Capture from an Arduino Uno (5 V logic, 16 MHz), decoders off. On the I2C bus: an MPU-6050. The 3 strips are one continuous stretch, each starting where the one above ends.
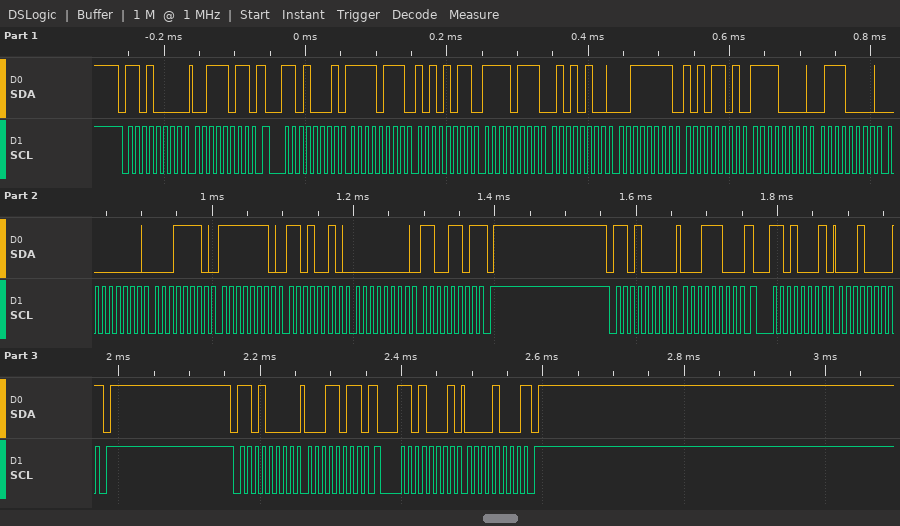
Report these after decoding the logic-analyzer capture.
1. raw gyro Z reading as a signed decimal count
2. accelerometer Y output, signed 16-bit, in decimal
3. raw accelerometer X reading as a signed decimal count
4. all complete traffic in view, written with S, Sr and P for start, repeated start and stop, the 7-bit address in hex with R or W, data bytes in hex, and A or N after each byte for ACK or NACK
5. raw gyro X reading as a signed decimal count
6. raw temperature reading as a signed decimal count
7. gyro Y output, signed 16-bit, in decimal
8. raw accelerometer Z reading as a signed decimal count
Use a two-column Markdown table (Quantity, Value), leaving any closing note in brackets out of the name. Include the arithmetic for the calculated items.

| Quantity | Value |
|---|---|
| raw gyro Z reading as a signed decimal count | 0x00CD = 205 |
| accelerometer Y output, signed 16-bit, in decimal | 0xF754 = -2220 |
| raw accelerometer X reading as a signed decimal count | 0xF7AB = -2133 |
| all complete traffic in view, written with S, Sr and P for start, repeated start and stop, the 7-bit address in hex with R or W, data bytes in hex, and A or N after each byte for ACK or NACK | S 68W A 3B A Sr 68R A F7 A AB A F7 A 54 A 3F A AD A F0 A 70 A 00 A 1E A FE A D2 A 00 A CD N P S 68W A 1C A Sr 68R A 10 N P S 68W A 1B A Sr 68R A 08 N P |
| raw gyro X reading as a signed decimal count | 0x001E = 30 |
| raw temperature reading as a signed decimal count | 0xF070 = -3984 |
| gyro Y output, signed 16-bit, in decimal | 0xFED2 = -302 |
| raw accelerometer Z reading as a signed decimal count | 0x3FAD = 16301 |
